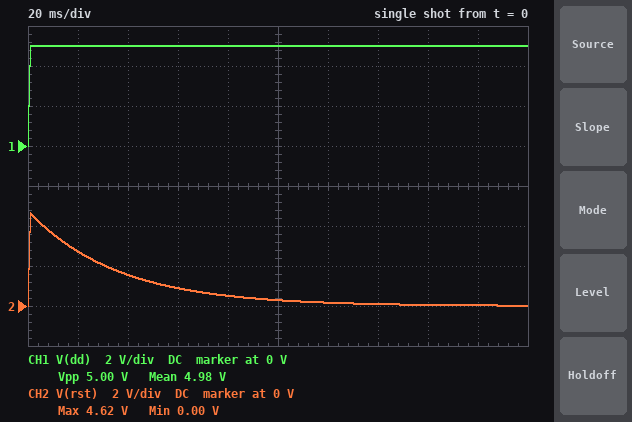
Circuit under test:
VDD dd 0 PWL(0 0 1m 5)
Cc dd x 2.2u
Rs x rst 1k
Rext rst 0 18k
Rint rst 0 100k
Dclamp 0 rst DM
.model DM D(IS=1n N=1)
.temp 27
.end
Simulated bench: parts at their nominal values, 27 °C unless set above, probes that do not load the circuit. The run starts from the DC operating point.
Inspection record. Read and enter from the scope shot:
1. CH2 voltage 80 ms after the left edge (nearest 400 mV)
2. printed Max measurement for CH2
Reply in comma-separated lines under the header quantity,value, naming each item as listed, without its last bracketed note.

quantity,value
CH2 voltage 80 ms after the left edge,400 mV
printed Max measurement for CH2,4.62 V
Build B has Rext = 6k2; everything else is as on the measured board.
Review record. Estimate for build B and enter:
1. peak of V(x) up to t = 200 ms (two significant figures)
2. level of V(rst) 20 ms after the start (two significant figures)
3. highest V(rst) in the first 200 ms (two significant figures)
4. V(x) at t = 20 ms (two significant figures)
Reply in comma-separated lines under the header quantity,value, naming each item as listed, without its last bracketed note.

quantity,value
peak of V(x) up to t = 200 ms,4.8 V
level of V(rst) 20 ms after the start,1.2 V
highest V(rst) in the first 200 ms,4.1 V
V(x) at t = 20 ms,1.4 V
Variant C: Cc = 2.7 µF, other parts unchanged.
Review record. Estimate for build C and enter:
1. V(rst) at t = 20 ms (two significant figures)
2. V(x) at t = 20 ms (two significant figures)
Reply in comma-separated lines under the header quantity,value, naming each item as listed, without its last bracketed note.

quantity,value
V(rst) at t = 20 ms,3.0 V
V(x) at t = 20 ms,3.2 V
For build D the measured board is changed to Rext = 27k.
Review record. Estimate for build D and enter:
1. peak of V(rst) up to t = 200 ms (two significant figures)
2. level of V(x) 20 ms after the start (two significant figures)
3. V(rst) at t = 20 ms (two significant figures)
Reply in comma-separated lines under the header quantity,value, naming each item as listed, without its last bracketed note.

quantity,value
peak of V(rst) up to t = 200 ms,4.7 V
level of V(x) 20 ms after the start,3.4 V
V(rst) at t = 20 ms,3.2 V
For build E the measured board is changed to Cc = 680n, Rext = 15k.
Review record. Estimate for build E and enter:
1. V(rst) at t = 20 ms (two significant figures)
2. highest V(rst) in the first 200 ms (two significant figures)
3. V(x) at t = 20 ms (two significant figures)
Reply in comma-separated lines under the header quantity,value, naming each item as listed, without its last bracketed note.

quantity,value
V(rst) at t = 20 ms,600 mV
highest V(rst) in the first 200 ms,4.4 V
V(x) at t = 20 ms,650 mV
